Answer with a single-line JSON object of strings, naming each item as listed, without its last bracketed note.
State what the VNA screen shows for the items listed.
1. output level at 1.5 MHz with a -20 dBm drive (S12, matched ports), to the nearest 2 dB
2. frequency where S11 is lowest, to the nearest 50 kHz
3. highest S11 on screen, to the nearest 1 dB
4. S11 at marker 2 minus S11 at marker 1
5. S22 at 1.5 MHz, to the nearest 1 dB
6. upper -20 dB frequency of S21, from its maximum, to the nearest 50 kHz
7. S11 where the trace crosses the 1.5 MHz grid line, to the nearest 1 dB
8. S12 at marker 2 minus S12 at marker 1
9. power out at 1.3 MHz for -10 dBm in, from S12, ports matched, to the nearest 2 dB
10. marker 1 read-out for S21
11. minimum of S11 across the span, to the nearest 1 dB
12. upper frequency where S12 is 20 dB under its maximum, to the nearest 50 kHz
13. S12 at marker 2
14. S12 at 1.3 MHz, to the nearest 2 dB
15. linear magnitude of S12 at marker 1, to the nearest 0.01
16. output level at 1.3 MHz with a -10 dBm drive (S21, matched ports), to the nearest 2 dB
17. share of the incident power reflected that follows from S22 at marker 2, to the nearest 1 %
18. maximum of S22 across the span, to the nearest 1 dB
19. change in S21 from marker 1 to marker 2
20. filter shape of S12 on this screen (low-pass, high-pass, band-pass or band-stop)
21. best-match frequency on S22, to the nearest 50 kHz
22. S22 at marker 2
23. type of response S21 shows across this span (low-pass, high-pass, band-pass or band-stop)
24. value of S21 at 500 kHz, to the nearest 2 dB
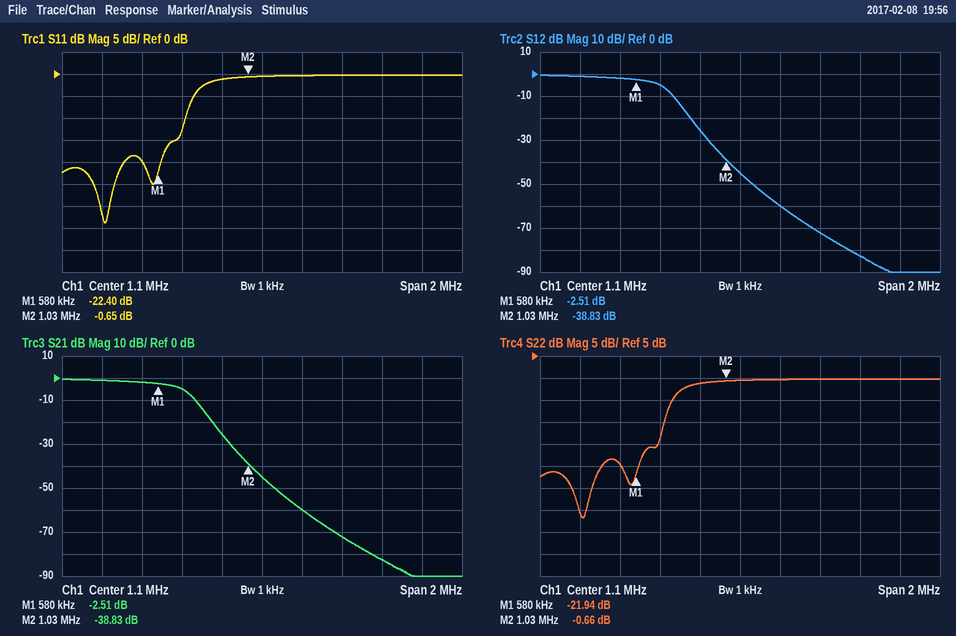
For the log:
{"output level at 1.5 MHz with a -20 dBm drive (S12, matched ports), to the nearest 2 dB": "-92 dBm", "frequency where S11 is lowest, to the nearest 50 kHz": "300 kHz", "highest S11 on screen, to the nearest 1 dB": "0 dB", "S11 at marker 2 minus S11 at marker 1": "21.75 dB", "S22 at 1.5 MHz, to the nearest 1 dB": "0 dB", "upper -20 dB frequency of S21, from its maximum, to the nearest 50 kHz": "850 kHz", "S11 where the trace crosses the 1.5 MHz grid line, to the nearest 1 dB": "0 dB", "S12 at marker 2 minus S12 at marker 1": "-36.32 dB", "power out at 1.3 MHz for -10 dBm in, from S12, ports matched, to the nearest 2 dB": "-70 dBm", "marker 1 read-out for S21": "-2.51 dB", "minimum of S11 across the span, to the nearest 1 dB": "-34 dB", "upper frequency where S12 is 20 dB under its maximum, to the nearest 50 kHz": "850 kHz", "S12 at marker 2": "-38.83 dB", "S12 at 1.3 MHz, to the nearest 2 dB": "-60 dB", "linear magnitude of S12 at marker 1, to the nearest 0.01": "0.75", "output level at 1.3 MHz with a -10 dBm drive (S21, matched ports), to the nearest 2 dB": "-70 dBm", "share of the incident power reflected that follows from S22 at marker 2, to the nearest 1 %": "86 %", "maximum of S22 across the span, to the nearest 1 dB": "0 dB", "change in S21 from marker 1 to marker 2": "-36.32 dB", "filter shape of S12 on this screen": "low-pass", "best-match frequency on S22, to the nearest 50 kHz": "300 kHz", "S22 at marker 2": "-0.66 dB", "type of response S21 shows across this span": "low-pass", "value of S21 at 500 kHz, to the nearest 2 dB": "-2 dB"}
